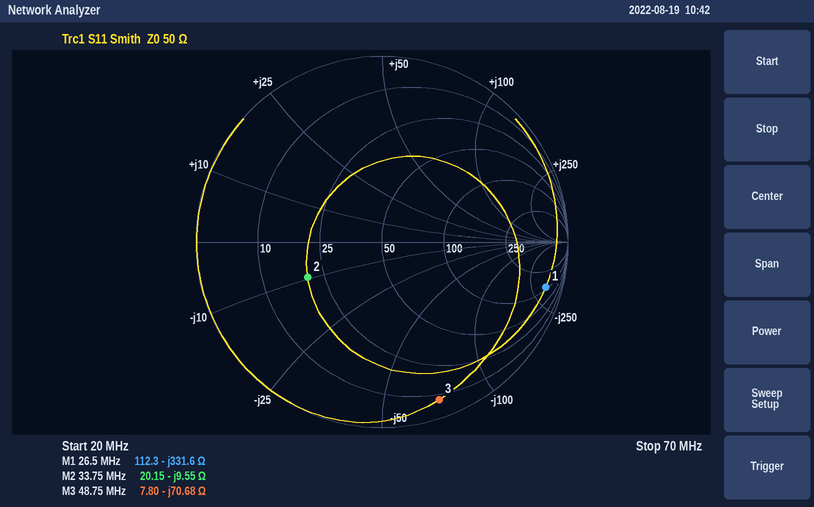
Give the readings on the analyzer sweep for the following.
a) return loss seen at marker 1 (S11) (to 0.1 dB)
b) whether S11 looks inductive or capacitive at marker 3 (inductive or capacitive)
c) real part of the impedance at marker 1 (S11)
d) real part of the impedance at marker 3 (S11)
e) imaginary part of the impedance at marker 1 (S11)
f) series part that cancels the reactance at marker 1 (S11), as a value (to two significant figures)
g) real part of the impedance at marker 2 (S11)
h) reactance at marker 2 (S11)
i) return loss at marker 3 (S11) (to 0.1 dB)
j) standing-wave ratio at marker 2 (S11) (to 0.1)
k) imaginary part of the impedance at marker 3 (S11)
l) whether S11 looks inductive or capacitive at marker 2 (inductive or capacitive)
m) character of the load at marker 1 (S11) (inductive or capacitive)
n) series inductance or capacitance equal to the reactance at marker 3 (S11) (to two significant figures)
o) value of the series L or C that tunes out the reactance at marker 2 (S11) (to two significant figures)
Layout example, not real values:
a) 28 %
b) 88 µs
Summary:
a) 0.8 dB
b) capacitive
c) 112.3 Ω
d) 7.80 Ω
e) -331.6 Ω
f) 2.0 µH
g) 20.15 Ω
h) -9.55 Ω
i) 0.9 dB
j) 2.6
k) -70.68 Ω
l) capacitive
m) capacitive
n) 46 pF
o) 45 nH
